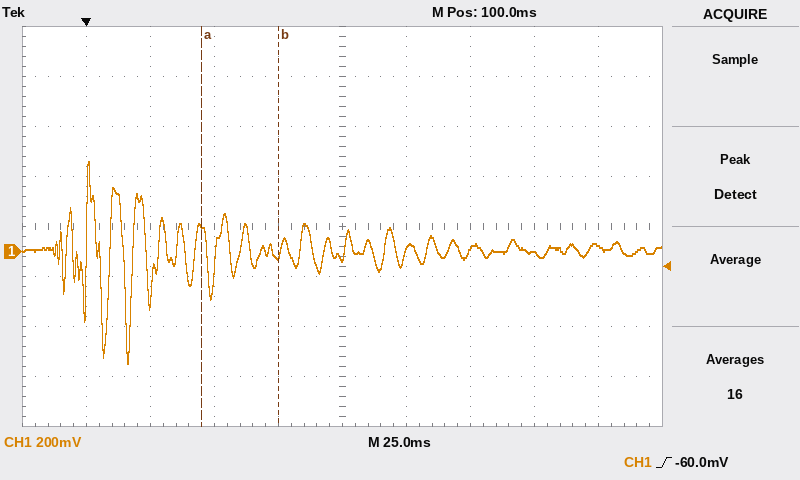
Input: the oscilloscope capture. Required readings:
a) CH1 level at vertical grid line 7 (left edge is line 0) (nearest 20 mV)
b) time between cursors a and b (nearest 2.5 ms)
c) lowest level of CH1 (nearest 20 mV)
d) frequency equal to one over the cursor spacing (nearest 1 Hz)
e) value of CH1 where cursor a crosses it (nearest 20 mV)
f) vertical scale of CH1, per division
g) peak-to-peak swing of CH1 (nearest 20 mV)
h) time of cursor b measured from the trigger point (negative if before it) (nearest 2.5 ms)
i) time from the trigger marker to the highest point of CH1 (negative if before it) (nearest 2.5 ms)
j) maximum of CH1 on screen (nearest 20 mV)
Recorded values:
0 mV
30.0 ms
-440 mV
33 Hz
100 mV
200 mV
800 mV
+75.0 ms
0.0 ms
360 mV
